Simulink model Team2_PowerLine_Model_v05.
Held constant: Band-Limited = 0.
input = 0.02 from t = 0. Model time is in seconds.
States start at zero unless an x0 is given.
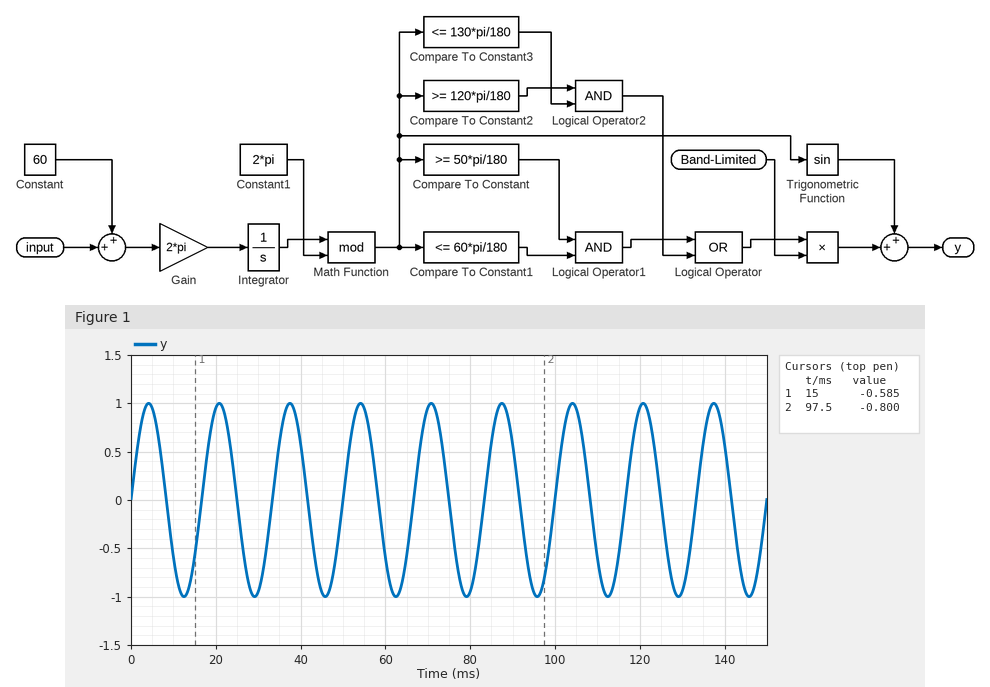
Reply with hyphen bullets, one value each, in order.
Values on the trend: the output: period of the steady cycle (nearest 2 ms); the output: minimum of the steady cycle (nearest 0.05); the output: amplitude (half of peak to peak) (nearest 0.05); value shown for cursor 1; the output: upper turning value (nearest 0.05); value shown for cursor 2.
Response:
- 16 ms
- -1.00
- 1.00
- -0.585
- 1.00
- -0.800
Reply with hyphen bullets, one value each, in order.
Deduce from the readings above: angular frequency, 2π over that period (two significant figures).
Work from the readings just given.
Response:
- 0.39 rad/ms
